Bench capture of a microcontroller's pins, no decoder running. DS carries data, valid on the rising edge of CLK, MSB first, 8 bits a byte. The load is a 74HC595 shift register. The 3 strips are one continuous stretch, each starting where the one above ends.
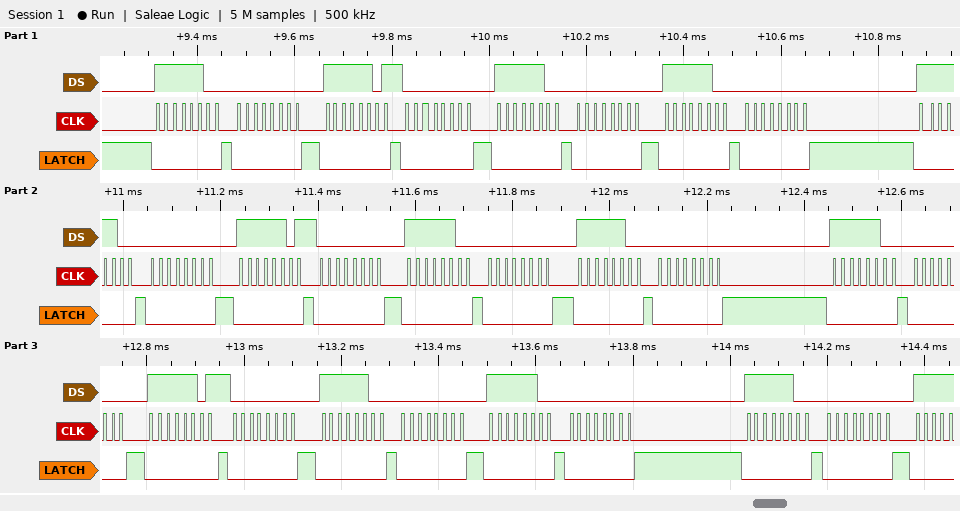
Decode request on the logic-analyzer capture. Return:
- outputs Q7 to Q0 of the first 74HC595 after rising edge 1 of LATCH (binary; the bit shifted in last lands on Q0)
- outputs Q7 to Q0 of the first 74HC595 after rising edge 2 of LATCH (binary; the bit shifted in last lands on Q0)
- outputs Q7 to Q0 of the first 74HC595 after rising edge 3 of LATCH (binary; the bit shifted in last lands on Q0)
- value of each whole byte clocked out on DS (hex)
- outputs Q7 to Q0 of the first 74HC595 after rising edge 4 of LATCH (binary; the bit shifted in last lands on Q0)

11111100
00000000
11111101
0xFC 0x00 0xFD 0x00 0xFC 0x00 0xFC 0x00 0xFC 0x00 0xFD 0x00 0xFC 0x00 0xFC 0x00 0xFC 0x00 0xFD 0x00 0xFC 0x00 0xFC 0x00 0xFC 0x00
00000000
